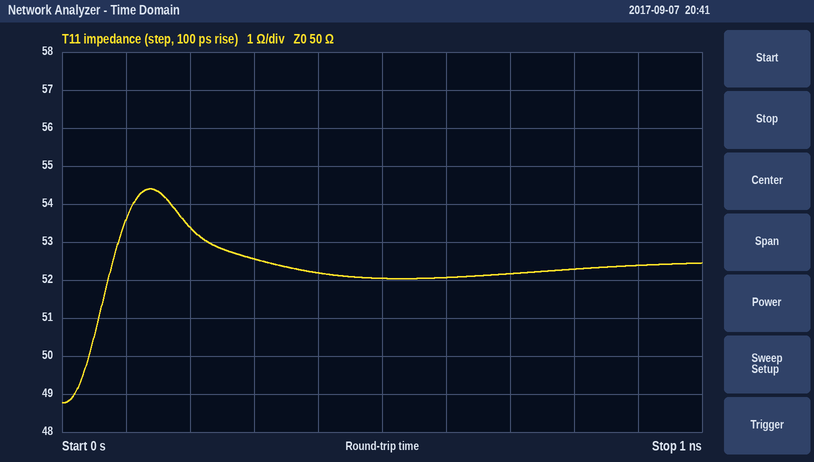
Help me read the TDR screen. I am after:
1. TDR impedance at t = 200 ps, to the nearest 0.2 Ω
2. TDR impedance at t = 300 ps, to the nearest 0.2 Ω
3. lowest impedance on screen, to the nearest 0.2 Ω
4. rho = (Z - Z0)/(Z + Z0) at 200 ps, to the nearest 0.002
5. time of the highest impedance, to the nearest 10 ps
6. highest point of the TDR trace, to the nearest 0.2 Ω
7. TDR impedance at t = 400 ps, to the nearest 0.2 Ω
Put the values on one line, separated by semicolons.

53.4 Ω; 52.6 Ω; 48.8 Ω; +0.032; 140 ps; 54.4 Ω; 52.2 Ω
